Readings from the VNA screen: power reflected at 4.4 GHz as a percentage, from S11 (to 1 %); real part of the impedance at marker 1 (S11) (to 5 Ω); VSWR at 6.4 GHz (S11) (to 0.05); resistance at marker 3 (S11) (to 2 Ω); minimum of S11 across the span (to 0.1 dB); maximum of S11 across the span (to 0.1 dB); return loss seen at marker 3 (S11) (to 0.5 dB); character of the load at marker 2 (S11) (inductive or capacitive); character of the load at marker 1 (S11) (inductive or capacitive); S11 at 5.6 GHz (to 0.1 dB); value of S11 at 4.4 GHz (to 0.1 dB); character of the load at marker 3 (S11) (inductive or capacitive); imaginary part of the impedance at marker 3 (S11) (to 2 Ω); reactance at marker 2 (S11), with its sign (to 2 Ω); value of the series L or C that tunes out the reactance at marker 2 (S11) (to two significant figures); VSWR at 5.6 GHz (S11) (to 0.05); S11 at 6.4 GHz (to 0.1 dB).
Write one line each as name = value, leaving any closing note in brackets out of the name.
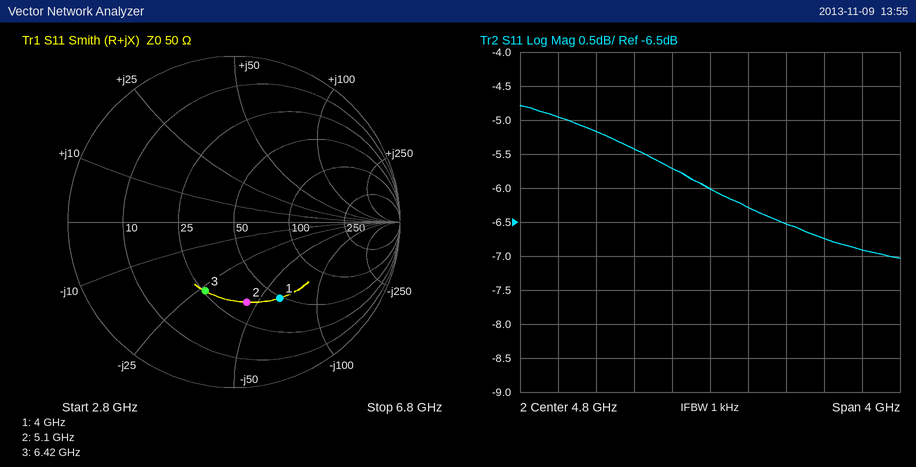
power reflected at 4.4 GHz as a percentage, from S11 = 27 %
real part of the impedance at marker 1 (S11) = 50 Ω
VSWR at 6.4 GHz (S11) = 2.65
resistance at marker 3 (S11) = 26 Ω
minimum of S11 across the span = -7.0 dB
maximum of S11 across the span = -4.8 dB
return loss seen at marker 3 (S11) = 7.0 dB
character of the load at marker 2 (S11) = capacitive
character of the load at marker 1 (S11) = capacitive
S11 at 5.6 GHz = -6.5 dB
value of S11 at 4.4 GHz = -5.7 dB
character of the load at marker 3 (S11) = capacitive
imaginary part of the impedance at marker 3 (S11) = -26 Ω
reactance at marker 2 (S11), with its sign = -44 Ω
value of the series L or C that tunes out the reactance at marker 2 (S11) = 1.4 nH
VSWR at 5.6 GHz (S11) = 2.80
S11 at 6.4 GHz = -6.9 dB
